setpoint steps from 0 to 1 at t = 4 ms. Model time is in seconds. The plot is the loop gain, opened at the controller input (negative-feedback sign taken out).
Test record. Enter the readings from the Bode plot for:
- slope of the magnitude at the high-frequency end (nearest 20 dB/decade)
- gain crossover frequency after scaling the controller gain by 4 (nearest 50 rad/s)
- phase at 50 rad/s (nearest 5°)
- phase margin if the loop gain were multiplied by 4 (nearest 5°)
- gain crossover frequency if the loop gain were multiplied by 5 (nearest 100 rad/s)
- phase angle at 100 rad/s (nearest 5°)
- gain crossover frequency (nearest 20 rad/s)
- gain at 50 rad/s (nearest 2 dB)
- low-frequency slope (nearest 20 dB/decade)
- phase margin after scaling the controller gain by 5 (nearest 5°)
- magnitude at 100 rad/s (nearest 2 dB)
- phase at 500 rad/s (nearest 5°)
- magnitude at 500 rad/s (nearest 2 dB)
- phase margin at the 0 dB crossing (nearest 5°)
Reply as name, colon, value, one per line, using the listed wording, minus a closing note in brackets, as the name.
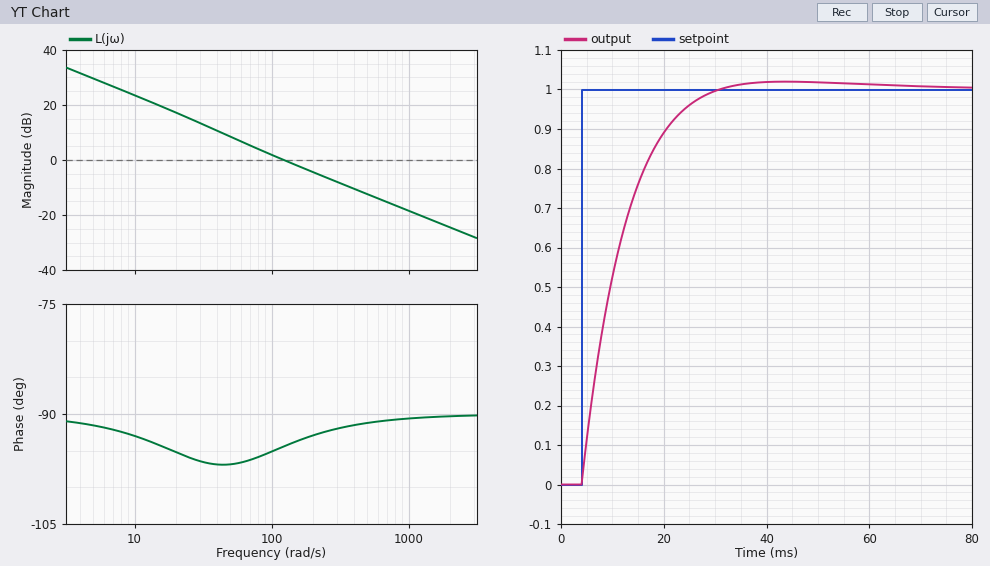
slope of the magnitude at the high-frequency end: -20 dB/decade
gain crossover frequency after scaling the controller gain by 4: 500 rad/s
phase at 50 rad/s: -95°
phase margin if the loop gain were multiplied by 4: 90°
gain crossover frequency if the loop gain were multiplied by 5: 600 rad/s
phase angle at 100 rad/s: -95°
gain crossover frequency: 120 rad/s
gain at 50 rad/s: 8 dB
low-frequency slope: -20 dB/decade
phase margin after scaling the controller gain by 5: 90°
magnitude at 100 rad/s: 2 dB
phase at 500 rad/s: -90°
magnitude at 500 rad/s: -12 dB
phase margin at the 0 dB crossing: 85°
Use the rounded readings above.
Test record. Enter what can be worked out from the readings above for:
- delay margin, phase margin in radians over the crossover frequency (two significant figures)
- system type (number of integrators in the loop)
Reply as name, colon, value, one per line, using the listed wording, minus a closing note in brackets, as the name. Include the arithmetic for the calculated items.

delay margin, phase margin in radians over the crossover frequency: 85 × π / 180 / 120 = 0.012 s
system type: 1
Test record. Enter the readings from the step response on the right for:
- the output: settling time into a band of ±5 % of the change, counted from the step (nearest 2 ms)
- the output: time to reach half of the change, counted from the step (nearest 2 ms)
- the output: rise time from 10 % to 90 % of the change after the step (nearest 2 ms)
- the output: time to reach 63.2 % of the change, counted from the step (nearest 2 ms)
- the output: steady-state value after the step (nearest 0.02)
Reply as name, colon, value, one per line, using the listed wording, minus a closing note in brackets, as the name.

the output: settling time into a band of ±5 % of the change, counted from the step: 20 ms
the output: time to reach half of the change, counted from the step: 6 ms
the output: rise time from 10 % to 90 % of the change after the step: 16 ms
the output: time to reach 63.2 % of the change, counted from the step: 8 ms
the output: steady-state value after the step: 1.00
